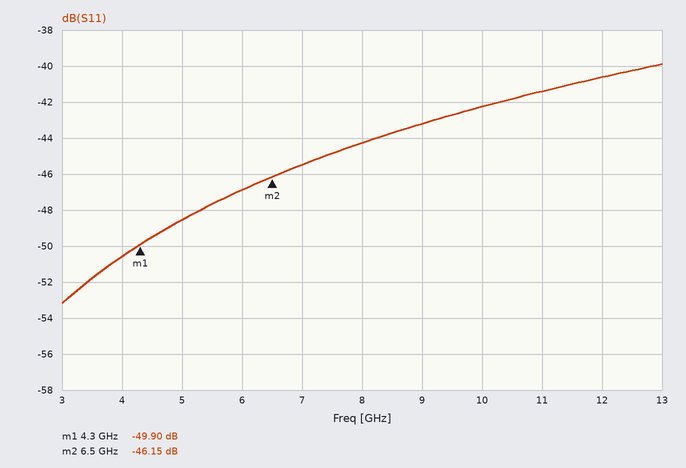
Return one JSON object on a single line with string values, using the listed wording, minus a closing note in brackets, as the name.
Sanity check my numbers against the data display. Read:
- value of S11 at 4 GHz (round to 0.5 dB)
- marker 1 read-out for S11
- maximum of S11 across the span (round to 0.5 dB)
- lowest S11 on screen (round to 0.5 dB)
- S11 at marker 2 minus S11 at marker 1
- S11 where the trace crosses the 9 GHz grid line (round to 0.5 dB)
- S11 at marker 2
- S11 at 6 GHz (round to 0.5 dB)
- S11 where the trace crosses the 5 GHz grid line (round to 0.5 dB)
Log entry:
{"value of S11 at 4 GHz": "-50.5 dB", "marker 1 read-out for S11": "-49.90 dB", "maximum of S11 across the span": "-40.0 dB", "lowest S11 on screen": "-53.0 dB", "S11 at marker 2 minus S11 at marker 1": "3.75 dB", "S11 where the trace crosses the 9 GHz grid line": "-43.0 dB", "S11 at marker 2": "-46.15 dB", "S11 at 6 GHz": "-47.0 dB", "S11 where the trace crosses the 5 GHz grid line": "-48.5 dB"}
